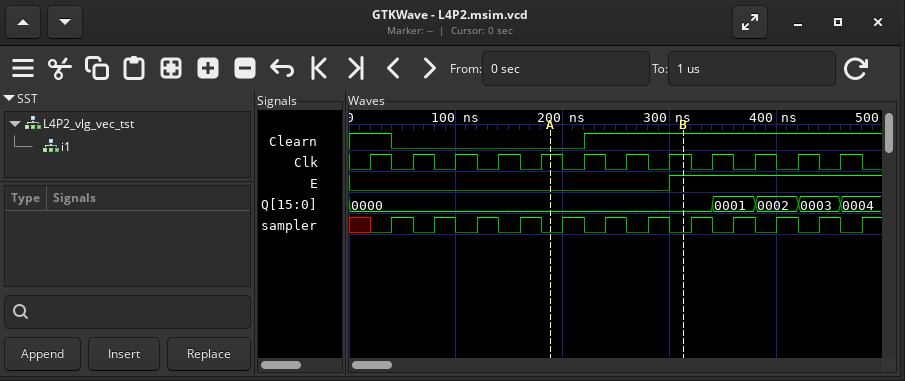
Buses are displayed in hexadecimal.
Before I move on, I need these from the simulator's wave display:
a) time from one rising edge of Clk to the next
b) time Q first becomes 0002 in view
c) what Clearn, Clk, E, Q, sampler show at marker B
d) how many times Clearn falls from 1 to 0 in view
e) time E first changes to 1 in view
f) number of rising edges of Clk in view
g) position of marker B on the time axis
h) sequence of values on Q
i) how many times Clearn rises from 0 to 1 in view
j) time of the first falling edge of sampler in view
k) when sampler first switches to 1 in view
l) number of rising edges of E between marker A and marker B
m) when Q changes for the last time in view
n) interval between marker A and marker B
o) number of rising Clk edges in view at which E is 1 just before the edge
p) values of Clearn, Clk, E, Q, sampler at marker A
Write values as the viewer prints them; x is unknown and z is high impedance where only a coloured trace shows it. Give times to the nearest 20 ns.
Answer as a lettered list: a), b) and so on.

a) 40 ns
b) 380 ns
c) Clearn=1, Clk=1, E=1, Q=0000, sampler=0
d) 1
e) 300 ns
f) 12
g) 320 ns
h) 0000, 0001, 0002, 0003, 0004
i) 1
j) 60 ns
k) 40 ns
l) 1
m) 460 ns
n) 120 ns
o) 4
p) Clearn=0, Clk=1, E=0, Q=0000, sampler=0
